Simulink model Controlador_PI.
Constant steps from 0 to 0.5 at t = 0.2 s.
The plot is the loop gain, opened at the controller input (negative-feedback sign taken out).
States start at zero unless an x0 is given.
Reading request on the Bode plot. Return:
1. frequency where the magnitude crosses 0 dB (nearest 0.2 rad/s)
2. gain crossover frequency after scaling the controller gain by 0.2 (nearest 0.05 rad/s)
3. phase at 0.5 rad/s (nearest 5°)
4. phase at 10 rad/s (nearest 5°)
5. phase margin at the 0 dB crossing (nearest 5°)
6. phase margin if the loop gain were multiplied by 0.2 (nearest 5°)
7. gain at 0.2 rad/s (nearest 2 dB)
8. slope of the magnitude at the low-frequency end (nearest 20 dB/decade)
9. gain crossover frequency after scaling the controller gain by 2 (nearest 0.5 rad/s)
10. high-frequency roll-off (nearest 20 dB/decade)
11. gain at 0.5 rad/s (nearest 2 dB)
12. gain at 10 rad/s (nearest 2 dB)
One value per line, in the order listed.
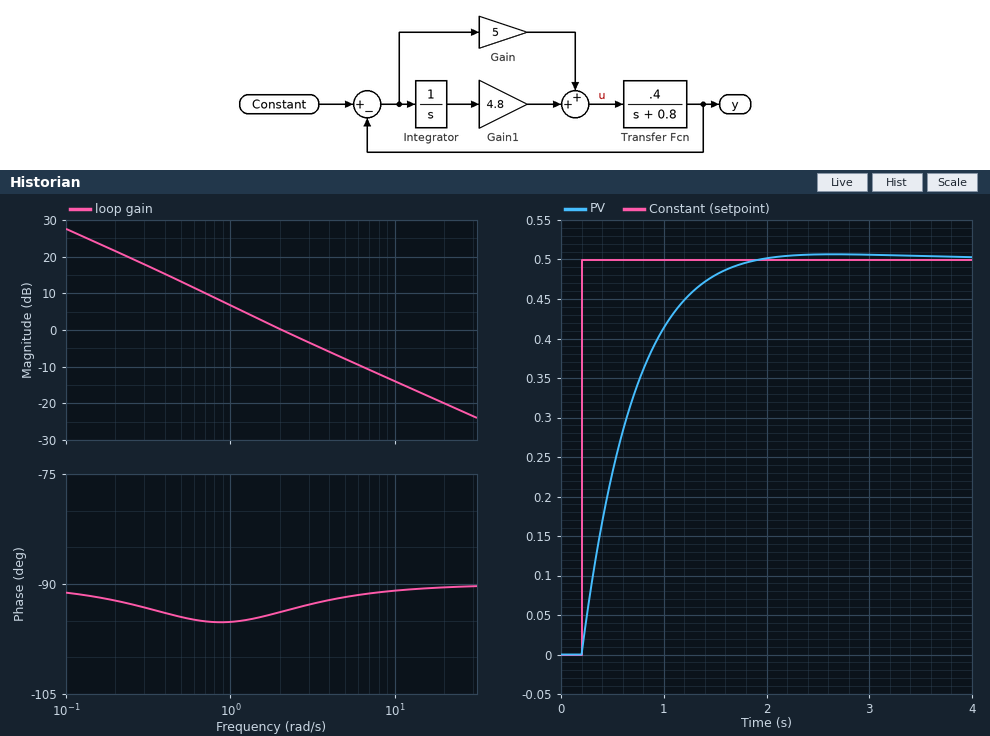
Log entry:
2.0 rad/s
0.45 rad/s
-95°
-90°
85°
85°
22 dB
-20 dB/decade
4.0 rad/s
-20 dB/decade
14 dB
-14 dB
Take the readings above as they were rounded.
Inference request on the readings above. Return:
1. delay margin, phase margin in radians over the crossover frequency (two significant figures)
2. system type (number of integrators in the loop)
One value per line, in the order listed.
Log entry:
0.74 s
1
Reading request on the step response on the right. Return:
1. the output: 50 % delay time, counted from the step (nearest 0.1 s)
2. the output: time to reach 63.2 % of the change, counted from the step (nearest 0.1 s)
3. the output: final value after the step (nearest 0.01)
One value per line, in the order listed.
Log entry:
0.3 s
0.5 s
0.50
